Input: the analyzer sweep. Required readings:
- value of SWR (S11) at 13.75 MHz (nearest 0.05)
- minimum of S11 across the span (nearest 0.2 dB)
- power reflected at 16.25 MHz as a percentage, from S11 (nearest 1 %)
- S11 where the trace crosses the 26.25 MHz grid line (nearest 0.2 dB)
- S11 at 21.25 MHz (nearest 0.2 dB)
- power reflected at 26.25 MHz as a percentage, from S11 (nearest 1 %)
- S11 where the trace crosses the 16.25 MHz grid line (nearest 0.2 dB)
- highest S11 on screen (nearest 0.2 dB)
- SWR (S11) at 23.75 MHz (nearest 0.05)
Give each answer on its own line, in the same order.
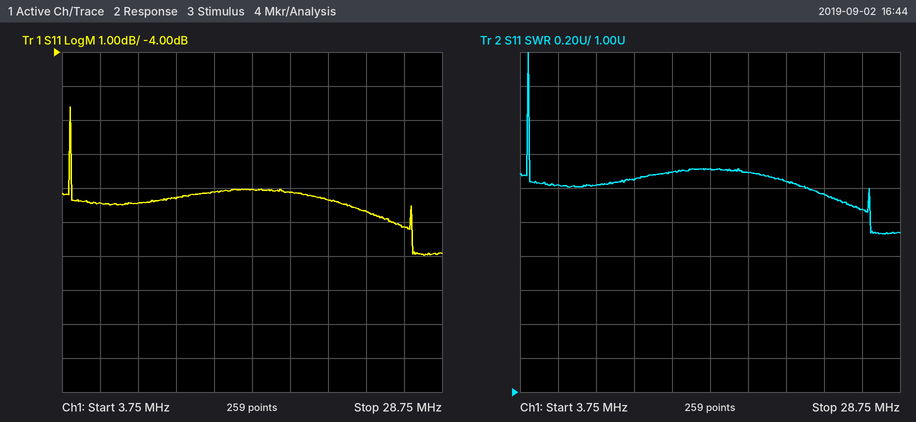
2.30
-10.0 dB
16 %
-9.2 dB
-8.4 dB
12 %
-8.0 dB
-5.6 dB
2.15
